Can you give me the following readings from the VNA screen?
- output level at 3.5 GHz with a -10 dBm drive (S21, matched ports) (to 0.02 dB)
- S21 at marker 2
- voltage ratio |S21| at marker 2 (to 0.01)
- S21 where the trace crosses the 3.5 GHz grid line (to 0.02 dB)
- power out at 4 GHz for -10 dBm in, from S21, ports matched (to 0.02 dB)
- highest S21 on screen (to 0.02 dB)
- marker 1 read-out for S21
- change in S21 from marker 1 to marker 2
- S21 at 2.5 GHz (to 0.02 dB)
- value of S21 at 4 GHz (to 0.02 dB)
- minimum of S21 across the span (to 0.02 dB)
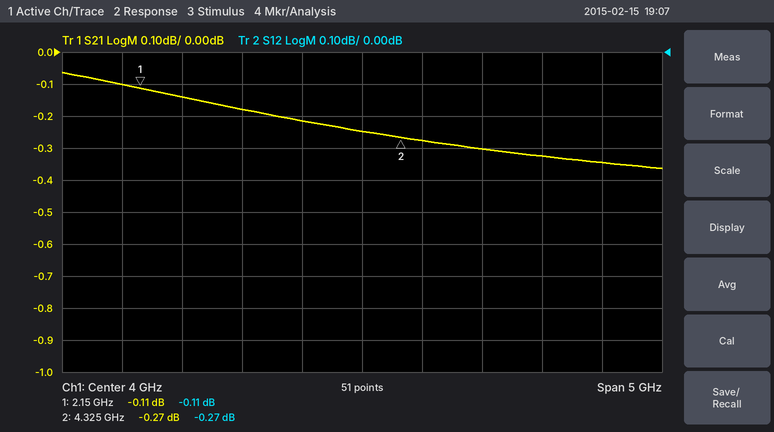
-10.22 dBm
-0.27 dB
0.97
-0.22 dB
-10.24 dBm
-0.06 dB
-0.11 dB
-0.16 dB
-0.14 dB
-0.24 dB
-0.36 dB
